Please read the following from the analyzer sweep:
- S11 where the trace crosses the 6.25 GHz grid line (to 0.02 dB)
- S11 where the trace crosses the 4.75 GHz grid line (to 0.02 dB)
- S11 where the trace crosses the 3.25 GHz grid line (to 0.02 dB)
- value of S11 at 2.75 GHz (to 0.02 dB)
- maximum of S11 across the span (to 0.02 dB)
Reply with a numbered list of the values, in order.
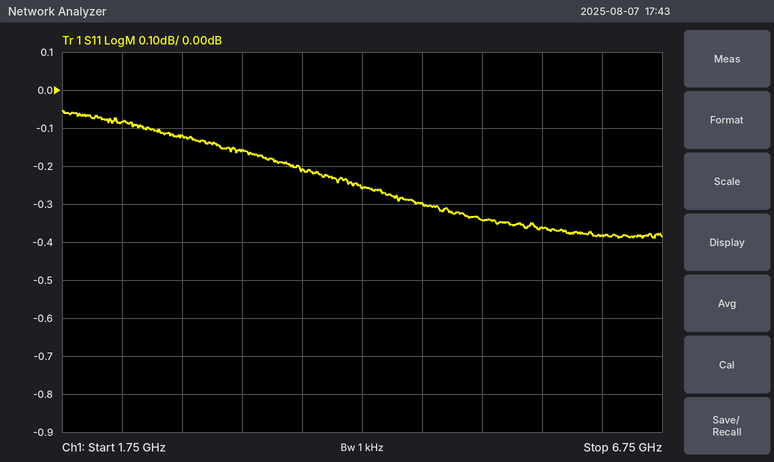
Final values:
1. -0.38 dB
2. -0.30 dB
3. -0.16 dB
4. -0.12 dB
5. -0.06 dB
